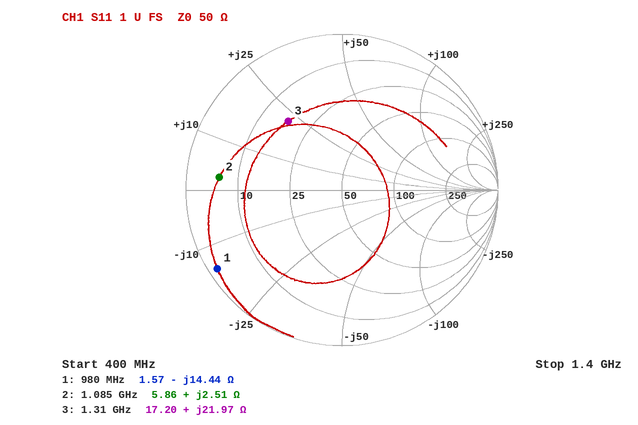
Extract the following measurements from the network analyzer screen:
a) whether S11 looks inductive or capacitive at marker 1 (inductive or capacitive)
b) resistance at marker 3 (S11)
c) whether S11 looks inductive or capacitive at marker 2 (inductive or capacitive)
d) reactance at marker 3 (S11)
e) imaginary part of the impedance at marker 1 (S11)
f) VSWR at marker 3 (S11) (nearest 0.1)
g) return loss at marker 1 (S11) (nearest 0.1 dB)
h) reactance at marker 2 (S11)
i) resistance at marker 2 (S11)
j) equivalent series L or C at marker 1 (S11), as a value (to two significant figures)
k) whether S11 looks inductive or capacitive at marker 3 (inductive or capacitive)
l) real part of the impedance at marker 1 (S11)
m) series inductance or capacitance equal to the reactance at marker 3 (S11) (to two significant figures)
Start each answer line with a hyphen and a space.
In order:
- capacitive
- 17.20 Ω
- inductive
- +21.97 Ω
- -14.44 Ω
- 3.5
- 0.5 dB
- +2.51 Ω
- 5.86 Ω
- 11 pF
- inductive
- 1.57 Ω
- 2.7 nH
